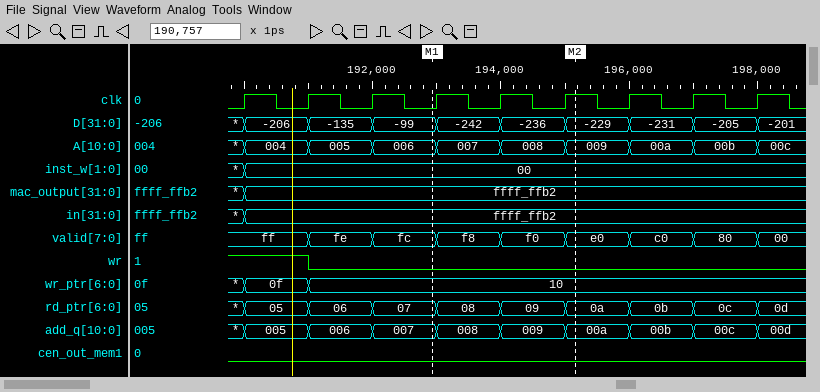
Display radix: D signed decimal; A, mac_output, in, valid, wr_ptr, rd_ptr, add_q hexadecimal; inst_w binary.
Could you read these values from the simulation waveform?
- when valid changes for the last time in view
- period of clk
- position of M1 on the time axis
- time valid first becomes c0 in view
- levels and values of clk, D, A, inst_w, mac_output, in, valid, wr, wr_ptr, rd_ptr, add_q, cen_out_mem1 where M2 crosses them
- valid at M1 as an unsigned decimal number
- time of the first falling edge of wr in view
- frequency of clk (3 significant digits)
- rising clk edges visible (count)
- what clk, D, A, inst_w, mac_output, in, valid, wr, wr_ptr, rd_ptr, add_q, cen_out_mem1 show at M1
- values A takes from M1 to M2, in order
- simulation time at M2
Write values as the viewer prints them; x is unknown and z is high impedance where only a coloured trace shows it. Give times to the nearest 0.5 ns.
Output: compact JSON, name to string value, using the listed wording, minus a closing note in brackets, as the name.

{"when valid changes for the last time in view": "198 ns", "period of clk": "1 ns", "position of M1 on the time axis": "193 ns", "time valid first becomes c0 in view": "196 ns", "levels and values of clk, D, A, inst_w, mac_output, in, valid, wr, wr_ptr, rd_ptr, add_q, cen_out_mem1 where M2 crosses them": "clk=1, D=-229, A=009, inst_w=00, mac_output=ffff_ffb2, in=ffff_ffb2, valid=e0, wr=0, wr_ptr=10, rd_ptr=0a, add_q=00a, cen_out_mem1=0", "valid at M1 as an unsigned decimal number": "252", "time of the first falling edge of wr in view": "191 ns", "frequency of clk": "1.00 GHz", "rising clk edges visible": "9", "what clk, D, A, inst_w, mac_output, in, valid, wr, wr_ptr, rd_ptr, add_q, cen_out_mem1 show at M1": "clk=0, D=-99, A=006, inst_w=00, mac_output=ffff_ffb2, in=ffff_ffb2, valid=fc, wr=0, wr_ptr=10, rd_ptr=07, add_q=007, cen_out_mem1=0", "values A takes from M1 to M2, in order": "006, 007, 008, 009", "simulation time at M2": "195 ns"}
